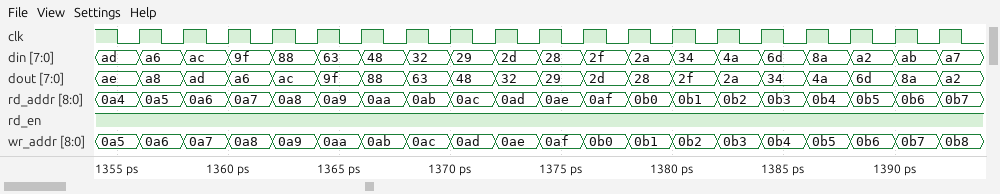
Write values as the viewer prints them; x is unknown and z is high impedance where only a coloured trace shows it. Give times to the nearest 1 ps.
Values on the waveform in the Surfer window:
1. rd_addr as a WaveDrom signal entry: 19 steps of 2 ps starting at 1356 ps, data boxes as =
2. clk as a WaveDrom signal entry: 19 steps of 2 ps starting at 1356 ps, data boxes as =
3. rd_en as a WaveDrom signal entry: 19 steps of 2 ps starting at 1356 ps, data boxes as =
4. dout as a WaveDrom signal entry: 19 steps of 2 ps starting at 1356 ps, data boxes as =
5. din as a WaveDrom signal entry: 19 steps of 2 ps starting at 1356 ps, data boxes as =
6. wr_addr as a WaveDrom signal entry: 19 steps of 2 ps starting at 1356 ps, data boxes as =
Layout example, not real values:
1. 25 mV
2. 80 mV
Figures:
1. {name: 'rd_addr', wave: '===================', data: '0a5 0a6 0a7 0a8 0a9 0aa 0ab 0ac 0ad 0ae 0af 0b0 0b1 0b2 0b3 0b4 0b5 0b6 0b7'}
2. {name: 'clk', wave: 'p..................'}
3. {name: 'rd_en', wave: '1..................'}
4. {name: 'dout', wave: '===================', data: 'a8 ad a6 ac 9f 88 63 48 32 29 2d 28 2f 2a 34 4a 6d 8a a2'}
5. {name: 'din', wave: '===================', data: 'a6 ac 9f 88 63 48 32 29 2d 28 2f 2a 34 4a 6d 8a a2 ab a7'}
6. {name: 'wr_addr', wave: '===================', data: '0a6 0a7 0a8 0a9 0aa 0ab 0ac 0ad 0ae 0af 0b0 0b1 0b2 0b3 0b4 0b5 0b6 0b7 0b8'}
